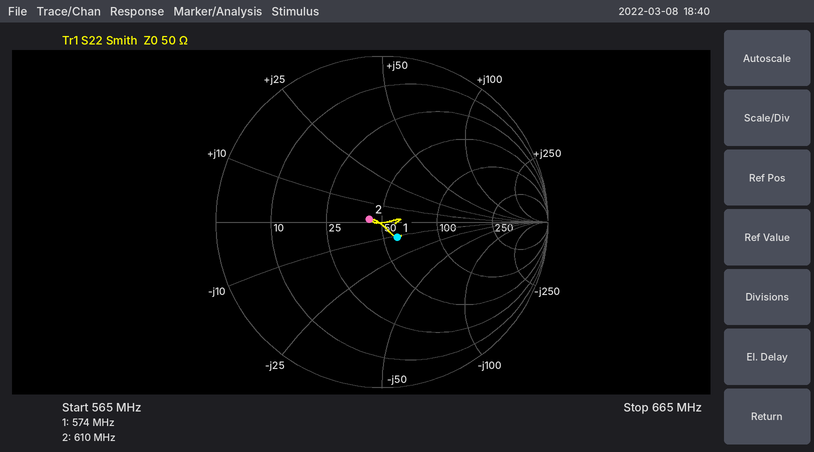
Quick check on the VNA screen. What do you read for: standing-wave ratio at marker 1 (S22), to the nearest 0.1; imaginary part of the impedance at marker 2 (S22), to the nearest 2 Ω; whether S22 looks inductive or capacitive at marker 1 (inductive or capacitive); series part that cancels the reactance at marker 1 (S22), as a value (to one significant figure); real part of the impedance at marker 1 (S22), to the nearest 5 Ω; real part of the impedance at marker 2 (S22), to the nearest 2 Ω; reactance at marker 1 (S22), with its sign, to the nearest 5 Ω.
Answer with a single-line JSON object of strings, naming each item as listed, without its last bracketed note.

{"standing-wave ratio at marker 1 (S22), to the nearest 0.1": "1.3", "imaginary part of the impedance at marker 2 (S22), to the nearest 2 Ω": "+2 Ω", "whether S22 looks inductive or capacitive at marker 1": "capacitive", "series part that cancels the reactance at marker 1 (S22), as a value": "3 nH", "real part of the impedance at marker 1 (S22), to the nearest 5 Ω": "60 Ω", "real part of the impedance at marker 2 (S22), to the nearest 2 Ω": "42 Ω", "reactance at marker 1 (S22), with its sign, to the nearest 5 Ω": "-10 Ω"}
